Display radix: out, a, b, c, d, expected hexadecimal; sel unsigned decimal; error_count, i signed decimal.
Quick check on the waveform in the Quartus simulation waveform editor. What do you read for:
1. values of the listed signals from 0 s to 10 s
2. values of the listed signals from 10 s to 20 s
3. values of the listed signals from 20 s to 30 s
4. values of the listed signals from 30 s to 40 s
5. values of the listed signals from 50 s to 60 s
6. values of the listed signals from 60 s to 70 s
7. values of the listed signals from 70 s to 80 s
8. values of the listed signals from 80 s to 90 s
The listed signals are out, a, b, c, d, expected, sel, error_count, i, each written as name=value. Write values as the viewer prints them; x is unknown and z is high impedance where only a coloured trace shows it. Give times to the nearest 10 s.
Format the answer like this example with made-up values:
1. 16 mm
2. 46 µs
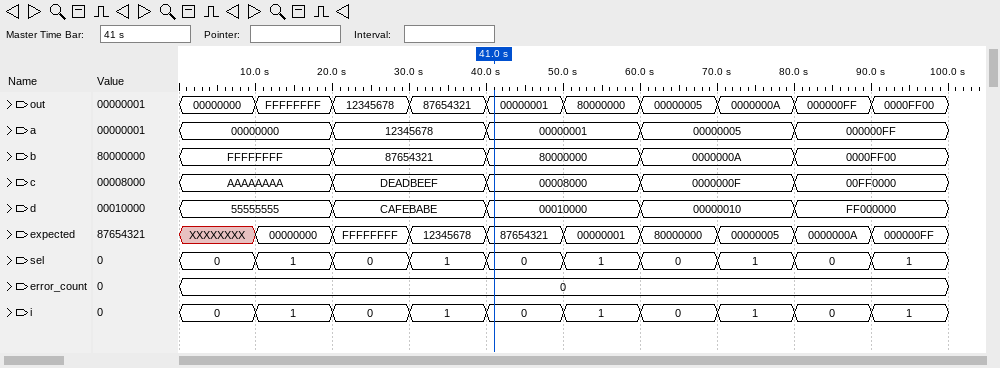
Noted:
1. out=00000000, a=00000000, b=FFFFFFFF, c=AAAAAAAA, d=55555555, expected=XXXXXXXX, sel=0, error_count=0, i=0
2. out=FFFFFFFF, a=00000000, b=FFFFFFFF, c=AAAAAAAA, d=55555555, expected=00000000, sel=1, error_count=0, i=1
3. out=12345678, a=12345678, b=87654321, c=DEADBEEF, d=CAFEBABE, expected=FFFFFFFF, sel=0, error_count=0, i=0
4. out=87654321, a=12345678, b=87654321, c=DEADBEEF, d=CAFEBABE, expected=12345678, sel=1, error_count=0, i=1
5. out=80000000, a=00000001, b=80000000, c=00008000, d=00010000, expected=00000001, sel=1, error_count=0, i=1
6. out=00000005, a=00000005, b=0000000A, c=0000000F, d=00000010, expected=80000000, sel=0, error_count=0, i=0
7. out=0000000A, a=00000005, b=0000000A, c=0000000F, d=00000010, expected=00000005, sel=1, error_count=0, i=1
8. out=000000FF, a=000000FF, b=0000FF00, c=00FF0000, d=FF000000, expected=0000000A, sel=0, error_count=0, i=0
